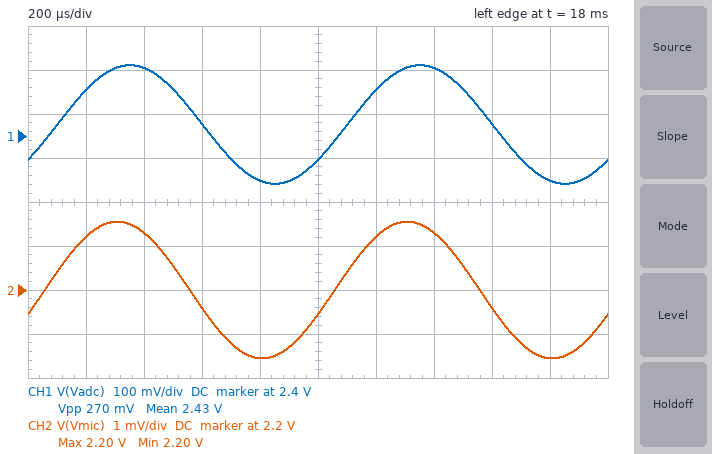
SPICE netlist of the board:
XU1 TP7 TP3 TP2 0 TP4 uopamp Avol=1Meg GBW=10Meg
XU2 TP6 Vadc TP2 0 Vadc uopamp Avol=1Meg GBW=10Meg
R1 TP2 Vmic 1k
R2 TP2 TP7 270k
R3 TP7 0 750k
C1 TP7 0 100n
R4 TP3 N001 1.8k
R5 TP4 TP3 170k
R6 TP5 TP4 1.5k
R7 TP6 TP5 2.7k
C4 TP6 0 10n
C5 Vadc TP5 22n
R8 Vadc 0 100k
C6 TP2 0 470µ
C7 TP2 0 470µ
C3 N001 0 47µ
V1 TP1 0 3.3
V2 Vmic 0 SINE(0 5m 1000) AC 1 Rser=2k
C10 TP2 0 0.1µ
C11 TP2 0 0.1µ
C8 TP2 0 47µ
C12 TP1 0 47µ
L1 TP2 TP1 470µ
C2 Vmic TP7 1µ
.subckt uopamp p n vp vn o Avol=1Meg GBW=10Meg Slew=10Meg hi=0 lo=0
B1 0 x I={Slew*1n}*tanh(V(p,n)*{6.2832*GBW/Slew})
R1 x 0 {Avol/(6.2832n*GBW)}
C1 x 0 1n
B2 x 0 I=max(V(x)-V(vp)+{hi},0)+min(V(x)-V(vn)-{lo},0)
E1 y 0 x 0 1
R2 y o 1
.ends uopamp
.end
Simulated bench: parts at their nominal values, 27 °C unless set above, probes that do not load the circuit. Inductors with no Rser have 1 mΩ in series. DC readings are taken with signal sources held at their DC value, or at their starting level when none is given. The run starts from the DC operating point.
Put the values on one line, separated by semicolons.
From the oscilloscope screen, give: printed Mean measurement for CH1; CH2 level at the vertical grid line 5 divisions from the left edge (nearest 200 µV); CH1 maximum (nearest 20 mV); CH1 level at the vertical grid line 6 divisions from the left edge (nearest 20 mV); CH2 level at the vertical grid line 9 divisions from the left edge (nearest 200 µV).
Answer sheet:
2.43 V; 2.1994 V; 2.56 V; 2.50 V; 2.1984 V
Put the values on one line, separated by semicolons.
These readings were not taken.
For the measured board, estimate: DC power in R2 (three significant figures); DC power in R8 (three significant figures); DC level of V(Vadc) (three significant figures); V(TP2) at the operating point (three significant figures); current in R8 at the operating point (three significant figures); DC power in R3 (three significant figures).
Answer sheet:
2.83 µW; 58.9 µW; 2.43 V; 3.30 V; 24.3 µA; 7.85 µW
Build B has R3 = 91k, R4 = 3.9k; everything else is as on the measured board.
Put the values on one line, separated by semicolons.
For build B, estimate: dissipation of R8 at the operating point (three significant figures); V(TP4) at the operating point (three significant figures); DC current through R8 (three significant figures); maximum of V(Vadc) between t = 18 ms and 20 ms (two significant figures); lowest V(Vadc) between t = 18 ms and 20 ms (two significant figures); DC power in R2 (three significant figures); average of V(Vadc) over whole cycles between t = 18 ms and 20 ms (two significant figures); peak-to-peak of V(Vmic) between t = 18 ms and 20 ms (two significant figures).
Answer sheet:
6.92 µW; 832 mV; 8.32 µA; 890 mV; 770 mV; 22.6 µW; 830 mV; 3.1 mV
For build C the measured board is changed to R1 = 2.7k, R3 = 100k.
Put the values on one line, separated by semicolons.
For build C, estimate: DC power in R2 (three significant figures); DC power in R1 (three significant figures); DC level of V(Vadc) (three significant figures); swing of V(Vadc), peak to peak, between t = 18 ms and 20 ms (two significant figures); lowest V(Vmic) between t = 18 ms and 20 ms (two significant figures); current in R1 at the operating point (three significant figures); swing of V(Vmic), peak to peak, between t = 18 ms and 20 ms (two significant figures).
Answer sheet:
21.5 µW; 1.33 mW; 892 mV; 410 mV; 1.4 V; 702 µA; 4.8 mV
